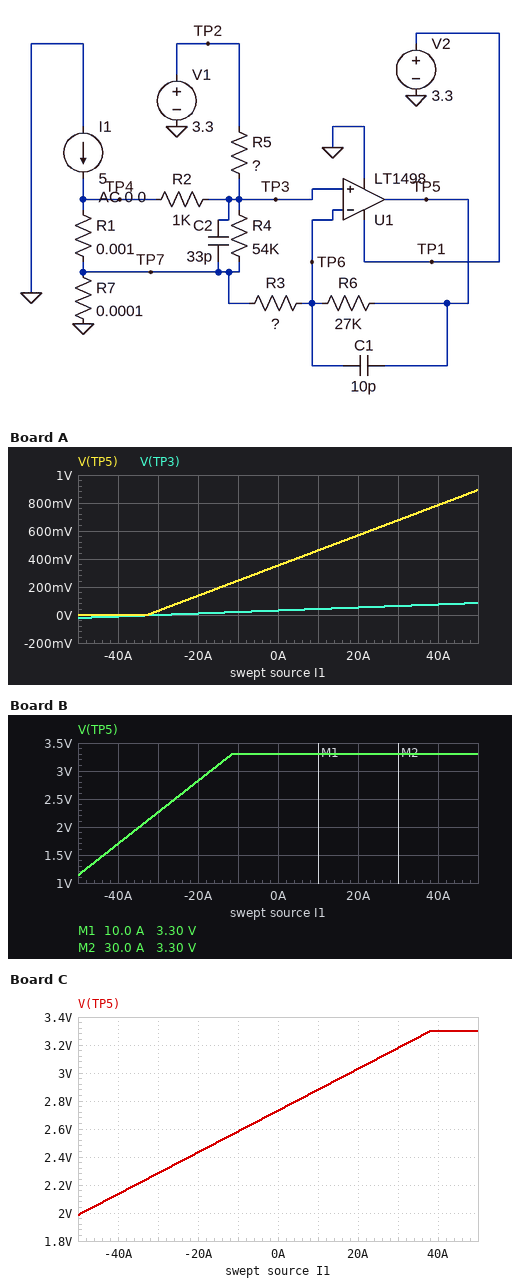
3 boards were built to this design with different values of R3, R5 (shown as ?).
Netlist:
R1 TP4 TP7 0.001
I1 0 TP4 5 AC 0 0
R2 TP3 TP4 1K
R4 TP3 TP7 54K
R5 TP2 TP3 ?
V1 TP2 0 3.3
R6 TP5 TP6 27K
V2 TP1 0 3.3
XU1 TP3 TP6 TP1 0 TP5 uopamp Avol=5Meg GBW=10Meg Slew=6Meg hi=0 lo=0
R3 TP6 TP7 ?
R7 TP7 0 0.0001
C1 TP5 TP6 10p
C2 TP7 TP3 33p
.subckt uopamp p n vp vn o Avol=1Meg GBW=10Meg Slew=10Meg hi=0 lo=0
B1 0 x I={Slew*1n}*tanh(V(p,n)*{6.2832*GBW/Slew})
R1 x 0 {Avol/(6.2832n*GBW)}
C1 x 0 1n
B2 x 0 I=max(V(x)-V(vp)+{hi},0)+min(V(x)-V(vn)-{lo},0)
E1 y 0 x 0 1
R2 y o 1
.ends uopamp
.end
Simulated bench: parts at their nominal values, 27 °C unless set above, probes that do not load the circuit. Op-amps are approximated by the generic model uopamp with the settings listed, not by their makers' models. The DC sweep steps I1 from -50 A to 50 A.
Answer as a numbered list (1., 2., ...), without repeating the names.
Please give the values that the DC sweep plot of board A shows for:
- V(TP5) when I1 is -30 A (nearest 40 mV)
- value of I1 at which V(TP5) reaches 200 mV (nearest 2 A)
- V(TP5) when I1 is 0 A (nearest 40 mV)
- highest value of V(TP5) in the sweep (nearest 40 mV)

1. 40 mV
2. -14 A
3. 360 mV
4. 880 mV
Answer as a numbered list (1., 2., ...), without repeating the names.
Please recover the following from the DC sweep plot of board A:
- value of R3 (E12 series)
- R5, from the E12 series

1. 2.7 kΩ
2. 100 kΩ
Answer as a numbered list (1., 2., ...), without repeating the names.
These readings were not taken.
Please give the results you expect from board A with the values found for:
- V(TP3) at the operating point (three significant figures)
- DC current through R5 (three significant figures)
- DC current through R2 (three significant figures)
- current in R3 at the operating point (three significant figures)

1. 37.4 mV
2. 32.6 µA
3. 31.9 µA
4. 13.7 µA
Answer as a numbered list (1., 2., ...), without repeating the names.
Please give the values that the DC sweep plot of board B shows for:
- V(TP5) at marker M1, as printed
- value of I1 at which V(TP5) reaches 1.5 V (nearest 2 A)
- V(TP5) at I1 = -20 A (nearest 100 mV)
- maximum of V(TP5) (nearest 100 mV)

1. 3.30 V
2. -44 A
3. 2.8 V
4. 3.3 V
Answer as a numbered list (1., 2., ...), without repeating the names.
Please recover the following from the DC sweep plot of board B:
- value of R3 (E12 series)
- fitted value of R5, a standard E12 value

1. 470 Ω
2. 47 kΩ
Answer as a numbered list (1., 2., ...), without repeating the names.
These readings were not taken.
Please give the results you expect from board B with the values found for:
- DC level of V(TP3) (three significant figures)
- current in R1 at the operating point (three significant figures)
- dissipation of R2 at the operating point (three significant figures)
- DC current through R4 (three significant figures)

1. 72.8 mV
2. 5.00 A
3. 4.53 µW
4. 1.34 µA
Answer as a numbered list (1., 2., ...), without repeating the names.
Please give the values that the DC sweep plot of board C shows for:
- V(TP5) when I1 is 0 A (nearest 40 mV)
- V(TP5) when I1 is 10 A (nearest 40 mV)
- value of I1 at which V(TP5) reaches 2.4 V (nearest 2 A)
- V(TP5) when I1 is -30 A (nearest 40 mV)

1. 2.72 V
2. 2.88 V
3. -22 A
4. 2.28 V
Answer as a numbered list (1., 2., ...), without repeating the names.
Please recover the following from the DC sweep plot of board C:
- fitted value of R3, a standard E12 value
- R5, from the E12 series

1. 1.8 kΩ
2. 18 kΩ
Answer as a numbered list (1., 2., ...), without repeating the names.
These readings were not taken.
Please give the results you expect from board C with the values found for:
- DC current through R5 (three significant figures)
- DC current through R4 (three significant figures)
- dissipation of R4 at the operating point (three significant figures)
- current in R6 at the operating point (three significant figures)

1. 174 µA
2. 3.25 µA
3. 569 nW
4. 97.4 µA
